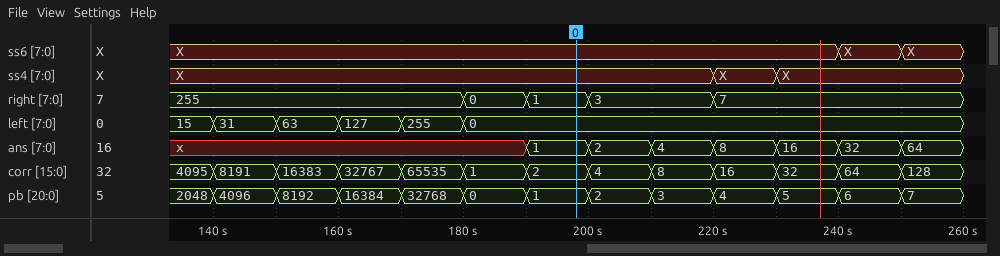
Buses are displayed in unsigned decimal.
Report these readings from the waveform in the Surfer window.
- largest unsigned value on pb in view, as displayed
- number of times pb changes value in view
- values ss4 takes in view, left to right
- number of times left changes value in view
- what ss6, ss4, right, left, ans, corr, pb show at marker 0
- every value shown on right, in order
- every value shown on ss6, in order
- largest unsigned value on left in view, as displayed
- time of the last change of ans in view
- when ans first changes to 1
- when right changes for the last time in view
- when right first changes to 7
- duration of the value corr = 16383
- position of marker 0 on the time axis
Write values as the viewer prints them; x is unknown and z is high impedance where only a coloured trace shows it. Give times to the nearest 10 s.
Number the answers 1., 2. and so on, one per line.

1. 32768
2. 12
3. X, X, X
4. 5
5. ss6=X, ss4=X, right=1, left=0, ans=1, corr=2, pb=1
6. 255, 0, 1, 3, 7
7. X, X, X
8. 255
9. 250 s
10. 190 s
11. 220 s
12. 220 s
13. 10 s
14. 200 s
